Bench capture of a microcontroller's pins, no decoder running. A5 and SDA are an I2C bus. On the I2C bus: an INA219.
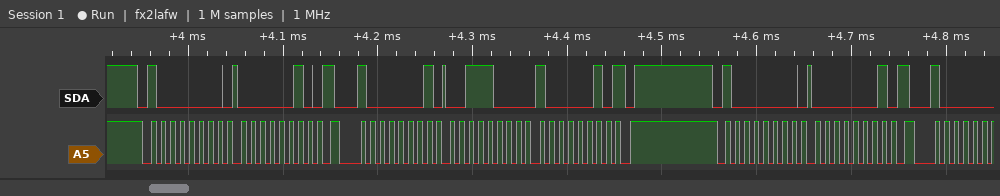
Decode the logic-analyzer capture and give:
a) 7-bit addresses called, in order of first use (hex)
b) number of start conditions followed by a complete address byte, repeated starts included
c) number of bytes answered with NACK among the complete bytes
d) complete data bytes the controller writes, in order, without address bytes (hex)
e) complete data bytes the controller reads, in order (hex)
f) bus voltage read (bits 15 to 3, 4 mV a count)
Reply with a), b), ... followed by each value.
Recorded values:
a) 0x40
b) 3
c) 1
d) 02 01
e) 38 82
f) 7.232 V
